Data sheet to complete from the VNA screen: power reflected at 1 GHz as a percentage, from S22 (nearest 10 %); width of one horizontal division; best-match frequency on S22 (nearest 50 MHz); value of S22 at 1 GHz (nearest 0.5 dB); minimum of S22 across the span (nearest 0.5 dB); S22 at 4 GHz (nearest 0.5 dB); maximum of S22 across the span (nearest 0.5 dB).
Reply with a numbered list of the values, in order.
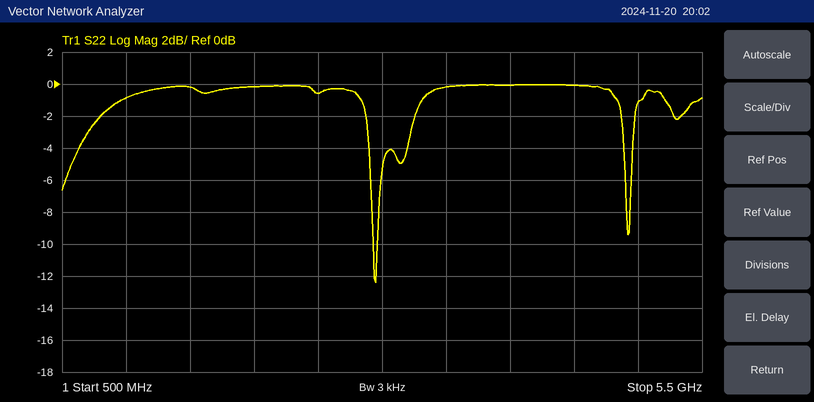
1. 80 %
2. 500 MHz
3. 2.95 GHz
4. -1.0 dB
5. -12.5 dB
6. 0.0 dB
7. 0.0 dB
